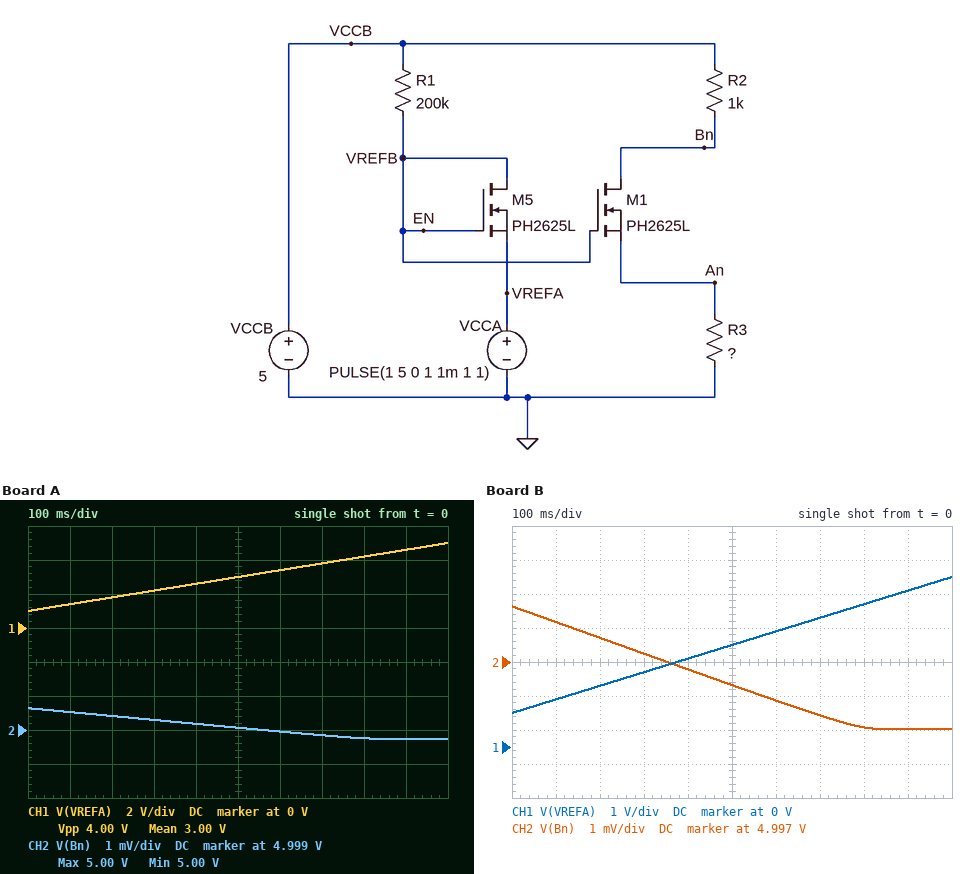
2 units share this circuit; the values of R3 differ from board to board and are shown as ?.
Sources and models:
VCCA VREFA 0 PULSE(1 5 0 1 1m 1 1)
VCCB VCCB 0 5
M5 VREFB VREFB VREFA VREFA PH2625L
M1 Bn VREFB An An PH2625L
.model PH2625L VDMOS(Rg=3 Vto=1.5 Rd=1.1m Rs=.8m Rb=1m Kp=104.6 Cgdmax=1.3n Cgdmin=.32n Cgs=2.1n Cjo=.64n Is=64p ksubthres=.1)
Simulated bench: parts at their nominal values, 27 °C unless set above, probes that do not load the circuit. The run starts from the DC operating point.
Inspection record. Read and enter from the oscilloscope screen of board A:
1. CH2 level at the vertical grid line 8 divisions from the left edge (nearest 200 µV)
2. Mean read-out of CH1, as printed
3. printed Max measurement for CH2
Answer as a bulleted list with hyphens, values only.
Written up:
- 4.9988 V
- 3.00 V
- 5.00 V
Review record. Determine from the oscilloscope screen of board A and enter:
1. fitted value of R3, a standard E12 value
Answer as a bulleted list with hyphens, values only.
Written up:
- 3.3 MΩ
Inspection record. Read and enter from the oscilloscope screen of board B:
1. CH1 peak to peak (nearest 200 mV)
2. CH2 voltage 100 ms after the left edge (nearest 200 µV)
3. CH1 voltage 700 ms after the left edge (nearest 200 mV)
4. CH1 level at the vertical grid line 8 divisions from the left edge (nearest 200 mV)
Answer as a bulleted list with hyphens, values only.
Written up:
- 4.0 V
- 4.9982 V
- 3.8 V
- 4.2 V
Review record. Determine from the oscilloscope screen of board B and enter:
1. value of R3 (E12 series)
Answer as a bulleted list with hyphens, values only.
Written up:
- 820 kΩ
